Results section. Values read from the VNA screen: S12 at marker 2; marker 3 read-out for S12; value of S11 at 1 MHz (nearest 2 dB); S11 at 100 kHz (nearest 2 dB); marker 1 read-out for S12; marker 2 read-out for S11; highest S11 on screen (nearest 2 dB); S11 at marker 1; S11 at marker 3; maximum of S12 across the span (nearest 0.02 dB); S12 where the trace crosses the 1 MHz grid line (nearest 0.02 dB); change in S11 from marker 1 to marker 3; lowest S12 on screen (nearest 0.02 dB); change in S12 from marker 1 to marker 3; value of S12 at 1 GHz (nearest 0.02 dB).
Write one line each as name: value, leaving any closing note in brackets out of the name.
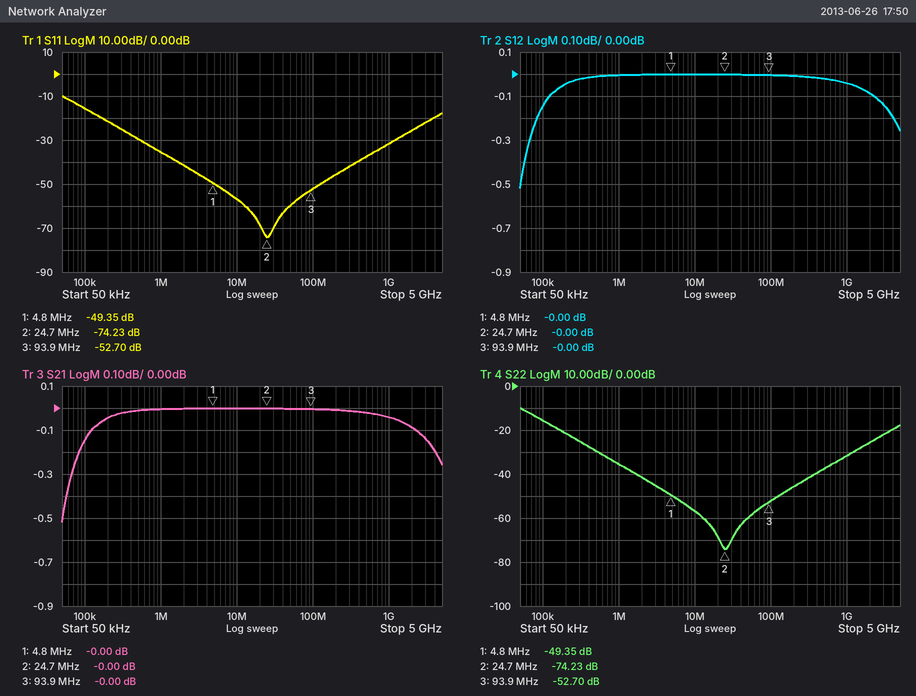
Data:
S12 at marker 2: -0.00 dB
marker 3 read-out for S12: -0.00 dB
value of S11 at 1 MHz: -36 dB
S11 at 100 kHz: -16 dB
marker 1 read-out for S12: -0.00 dB
marker 2 read-out for S11: -74.23 dB
highest S11 on screen: -10 dB
S11 at marker 1: -49.35 dB
S11 at marker 3: -52.70 dB
maximum of S12 across the span: 0.00 dB
S12 where the trace crosses the 1 MHz grid line: 0.00 dB
change in S11 from marker 1 to marker 3: -3.35 dB
lowest S12 on screen: -0.52 dB
change in S12 from marker 1 to marker 3: 0.00 dB
value of S12 at 1 GHz: -0.04 dB
